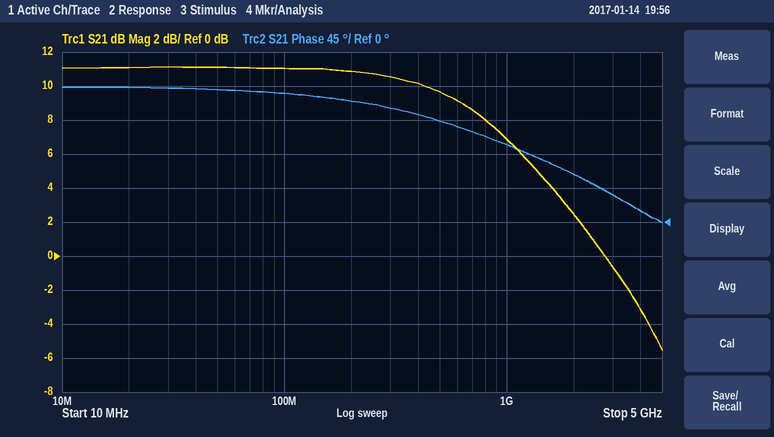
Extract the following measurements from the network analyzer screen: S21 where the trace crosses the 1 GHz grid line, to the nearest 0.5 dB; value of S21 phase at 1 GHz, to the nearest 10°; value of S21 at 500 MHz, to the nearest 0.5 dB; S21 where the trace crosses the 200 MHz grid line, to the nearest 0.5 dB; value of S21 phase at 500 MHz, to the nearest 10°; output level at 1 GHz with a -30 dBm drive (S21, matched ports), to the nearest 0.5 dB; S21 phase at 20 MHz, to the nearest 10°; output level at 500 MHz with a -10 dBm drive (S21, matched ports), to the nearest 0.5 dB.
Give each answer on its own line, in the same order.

7.0 dB
100°
9.5 dB
11.0 dB
130°
-23.0 dBm
180°
-0.5 dBm
